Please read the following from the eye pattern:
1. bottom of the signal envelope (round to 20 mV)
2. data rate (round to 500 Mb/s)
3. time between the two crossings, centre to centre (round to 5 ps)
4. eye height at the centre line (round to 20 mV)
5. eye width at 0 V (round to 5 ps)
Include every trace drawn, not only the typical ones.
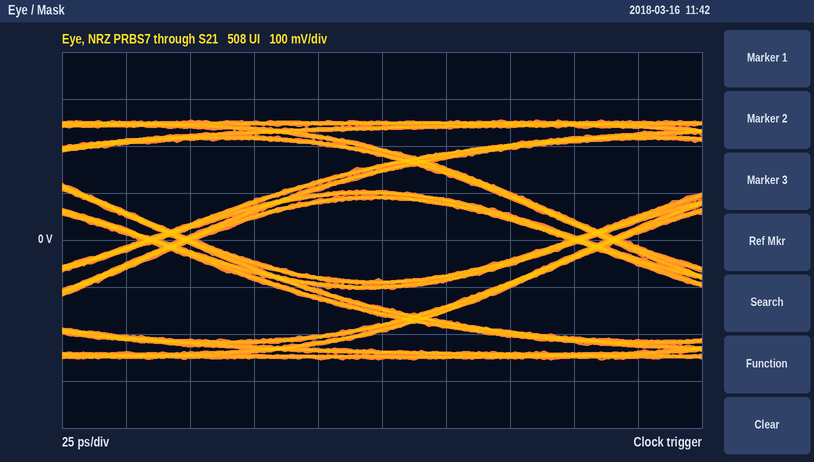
-260 mV
6.0 Gb/s
165 ps
180 mV
145 ps
